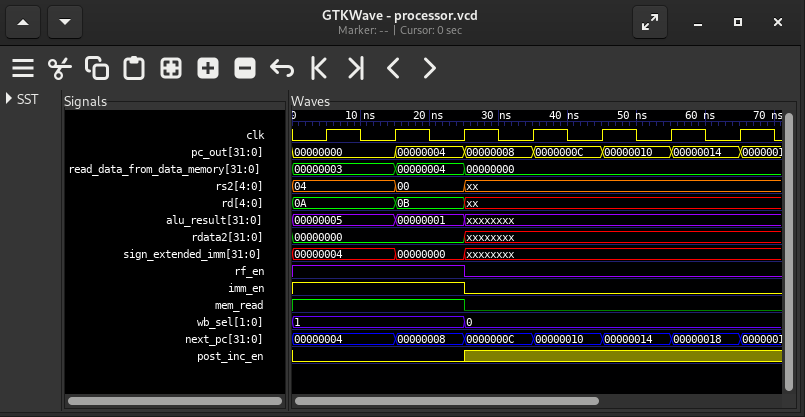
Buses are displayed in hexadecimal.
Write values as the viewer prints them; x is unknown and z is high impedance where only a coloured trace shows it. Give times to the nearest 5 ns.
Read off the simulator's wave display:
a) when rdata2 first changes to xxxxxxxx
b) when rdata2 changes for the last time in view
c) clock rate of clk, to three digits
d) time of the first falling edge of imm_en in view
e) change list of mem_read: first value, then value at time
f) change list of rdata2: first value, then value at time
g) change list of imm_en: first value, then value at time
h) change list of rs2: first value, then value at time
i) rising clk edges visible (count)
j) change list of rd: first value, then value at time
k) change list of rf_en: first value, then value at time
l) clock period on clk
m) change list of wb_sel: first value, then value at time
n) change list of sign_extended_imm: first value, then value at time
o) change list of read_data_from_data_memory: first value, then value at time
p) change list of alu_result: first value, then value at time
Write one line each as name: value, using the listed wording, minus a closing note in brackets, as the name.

when rdata2 first changes to xxxxxxxx: 25 ns
when rdata2 changes for the last time in view: 25 ns
clock rate of clk, to three digits: 100 MHz
time of the first falling edge of imm_en in view: 25 ns
change list of mem_read: first value, then value at time: 1, 0 at 25 ns
change list of rdata2: first value, then value at time: 00000000, xxxxxxxx at 25 ns
change list of imm_en: first value, then value at time: 1, 0 at 25 ns
change list of rs2: first value, then value at time: 04, 00 at 15 ns, xx at 25 ns
rising clk edges visible: 7
change list of rd: first value, then value at time: 0A, 0B at 15 ns, xx at 25 ns
change list of rf_en: first value, then value at time: 1, 0 at 25 ns
clock period on clk: 10 ns
change list of wb_sel: first value, then value at time: 1, 0 at 25 ns
change list of sign_extended_imm: first value, then value at time: 00000004, 00000000 at 15 ns, xxxxxxxx at 25 ns
change list of read_data_from_data_memory: first value, then value at time: 00000003, 00000004 at 15 ns, 00000000 at 25 ns
change list of alu_result: first value, then value at time: 00000005, 00000001 at 15 ns, xxxxxxxx at 25 ns
